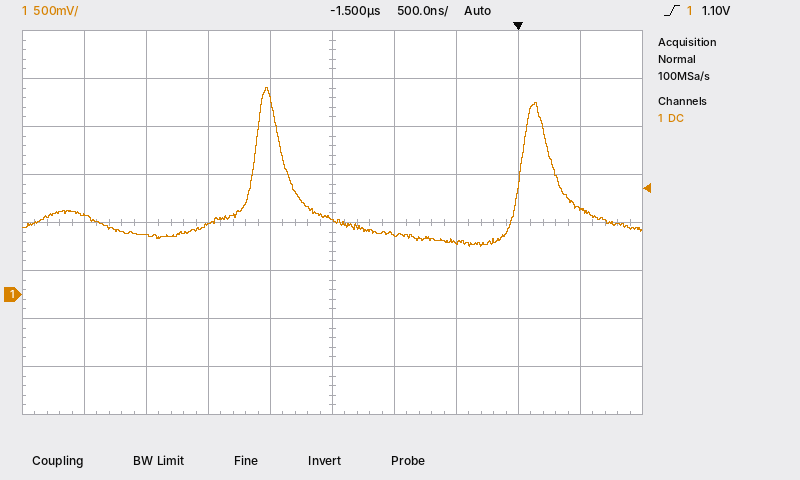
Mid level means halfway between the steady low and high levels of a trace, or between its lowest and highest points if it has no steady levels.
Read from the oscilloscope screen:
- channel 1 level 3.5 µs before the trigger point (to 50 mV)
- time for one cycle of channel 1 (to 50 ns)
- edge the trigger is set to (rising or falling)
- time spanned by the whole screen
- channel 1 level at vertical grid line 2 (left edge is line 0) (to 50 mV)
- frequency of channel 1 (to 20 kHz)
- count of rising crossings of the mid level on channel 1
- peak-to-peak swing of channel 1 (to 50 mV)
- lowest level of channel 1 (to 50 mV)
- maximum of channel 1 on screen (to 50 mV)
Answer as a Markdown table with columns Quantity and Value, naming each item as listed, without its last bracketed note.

| Quantity | Value |
|---|---|
| channel 1 level 3.5 µs before the trigger point | 850 mV |
| time for one cycle of channel 1 | 2.15 µs |
| edge the trigger is set to | rising |
| time spanned by the whole screen | 5 µs |
| channel 1 level at vertical grid line 2 (left edge is line 0) | 600 mV |
| frequency of channel 1 | 460 kHz |
| count of rising crossings of the mid level on channel 1 | 2 |
| peak-to-peak swing of channel 1 | 1.65 V |
| lowest level of channel 1 | 500 mV |
| maximum of channel 1 on screen | 2.15 V |
